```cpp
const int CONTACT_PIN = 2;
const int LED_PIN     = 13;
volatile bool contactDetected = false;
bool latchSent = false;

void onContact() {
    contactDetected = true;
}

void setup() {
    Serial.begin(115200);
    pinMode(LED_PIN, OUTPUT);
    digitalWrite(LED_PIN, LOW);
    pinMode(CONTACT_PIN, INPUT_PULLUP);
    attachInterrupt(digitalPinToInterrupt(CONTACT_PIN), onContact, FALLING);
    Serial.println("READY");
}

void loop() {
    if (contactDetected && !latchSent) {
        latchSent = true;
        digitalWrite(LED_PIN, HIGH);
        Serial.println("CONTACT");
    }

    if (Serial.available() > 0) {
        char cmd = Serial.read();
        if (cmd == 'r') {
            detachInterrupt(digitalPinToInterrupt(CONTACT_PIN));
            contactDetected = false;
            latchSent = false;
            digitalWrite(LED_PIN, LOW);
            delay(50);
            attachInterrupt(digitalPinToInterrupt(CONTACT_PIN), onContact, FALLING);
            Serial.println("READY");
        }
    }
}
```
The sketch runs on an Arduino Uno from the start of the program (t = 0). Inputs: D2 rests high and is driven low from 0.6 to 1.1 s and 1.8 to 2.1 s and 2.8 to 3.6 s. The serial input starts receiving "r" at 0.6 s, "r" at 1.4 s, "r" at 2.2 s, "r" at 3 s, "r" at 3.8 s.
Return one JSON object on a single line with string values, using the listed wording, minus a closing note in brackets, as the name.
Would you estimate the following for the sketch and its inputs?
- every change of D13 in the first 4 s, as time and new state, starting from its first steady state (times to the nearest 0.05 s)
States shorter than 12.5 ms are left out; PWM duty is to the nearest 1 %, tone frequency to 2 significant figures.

{"every change of D13 in the first 4 s, as time and new state, starting from its first steady state": "0 s low; 1.8 s high; 2.2 s low; 2.8 s high; 3 s low"}
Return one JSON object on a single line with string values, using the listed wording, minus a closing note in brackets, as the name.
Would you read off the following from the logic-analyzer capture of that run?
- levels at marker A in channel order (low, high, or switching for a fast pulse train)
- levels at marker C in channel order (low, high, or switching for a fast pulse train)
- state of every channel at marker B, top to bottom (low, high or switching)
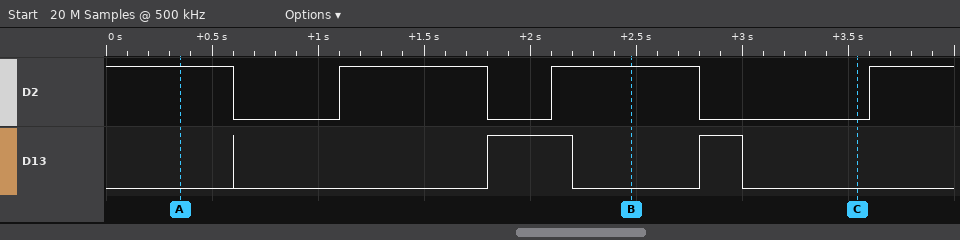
{"levels at marker A in channel order": "D2 high, D13 low", "levels at marker C in channel order": "D2 low, D13 low", "state of every channel at marker B, top to bottom": "D2 high, D13 low"}
